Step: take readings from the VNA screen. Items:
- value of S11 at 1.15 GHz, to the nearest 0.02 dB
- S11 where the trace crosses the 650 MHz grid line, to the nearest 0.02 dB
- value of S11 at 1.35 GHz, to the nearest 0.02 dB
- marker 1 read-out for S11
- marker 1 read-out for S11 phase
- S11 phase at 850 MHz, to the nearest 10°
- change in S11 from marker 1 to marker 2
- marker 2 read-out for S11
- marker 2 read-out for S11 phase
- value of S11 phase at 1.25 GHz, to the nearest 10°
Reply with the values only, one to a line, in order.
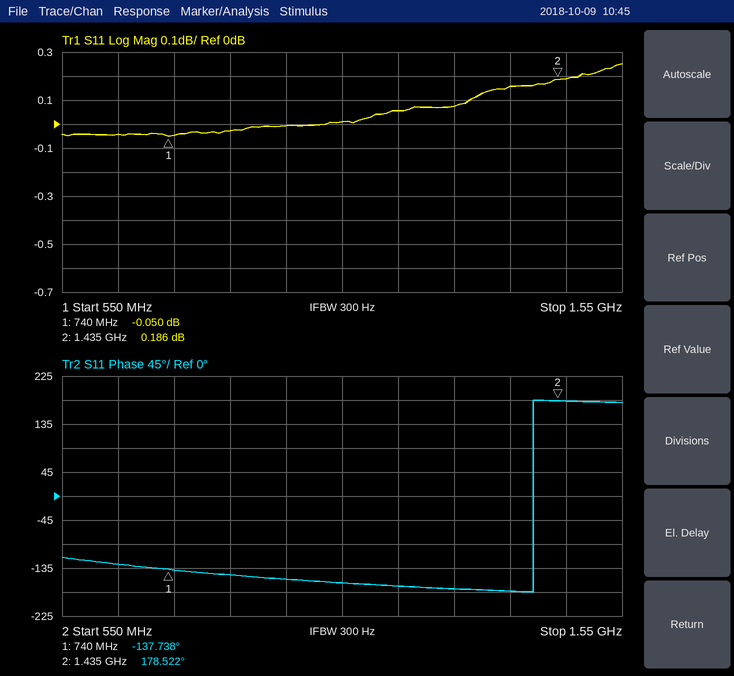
0.06 dB
-0.04 dB
0.16 dB
-0.050 dB
-137.738°
-150°
0.236 dB
0.186 dB
178.522°
-170°
